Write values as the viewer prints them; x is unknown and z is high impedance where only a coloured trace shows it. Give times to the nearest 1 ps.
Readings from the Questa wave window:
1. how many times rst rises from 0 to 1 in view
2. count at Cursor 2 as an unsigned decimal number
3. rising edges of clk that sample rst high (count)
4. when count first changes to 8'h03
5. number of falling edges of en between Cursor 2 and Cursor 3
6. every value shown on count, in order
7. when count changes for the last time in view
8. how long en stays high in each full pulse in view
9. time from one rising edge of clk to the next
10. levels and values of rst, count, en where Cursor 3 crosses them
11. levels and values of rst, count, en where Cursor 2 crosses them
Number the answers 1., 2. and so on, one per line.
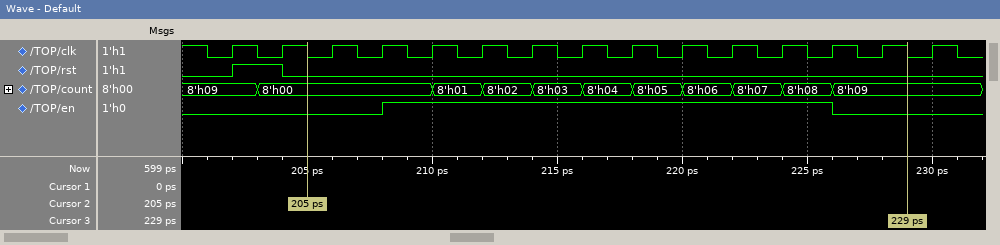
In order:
1. 1
2. 0
3. 1
4. 214 ps
5. 1
6. 8'h09, 8'h00, 8'h01, 8'h02, 8'h03, 8'h04, 8'h05, 8'h06, 8'h07, 8'h08, 8'h09
7. 226 ps
8. 18 ps
9. 2 ps
10. rst=0, count=8'h09, en=0
11. rst=0, count=8'h00, en=0
